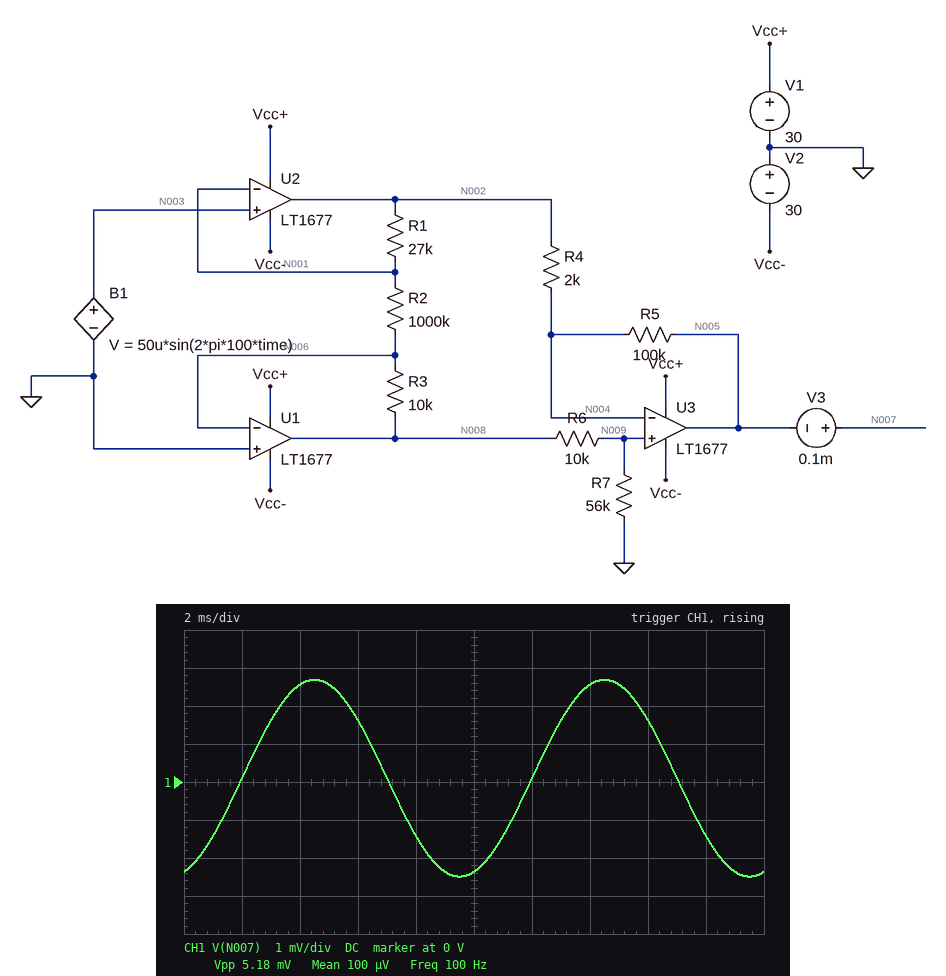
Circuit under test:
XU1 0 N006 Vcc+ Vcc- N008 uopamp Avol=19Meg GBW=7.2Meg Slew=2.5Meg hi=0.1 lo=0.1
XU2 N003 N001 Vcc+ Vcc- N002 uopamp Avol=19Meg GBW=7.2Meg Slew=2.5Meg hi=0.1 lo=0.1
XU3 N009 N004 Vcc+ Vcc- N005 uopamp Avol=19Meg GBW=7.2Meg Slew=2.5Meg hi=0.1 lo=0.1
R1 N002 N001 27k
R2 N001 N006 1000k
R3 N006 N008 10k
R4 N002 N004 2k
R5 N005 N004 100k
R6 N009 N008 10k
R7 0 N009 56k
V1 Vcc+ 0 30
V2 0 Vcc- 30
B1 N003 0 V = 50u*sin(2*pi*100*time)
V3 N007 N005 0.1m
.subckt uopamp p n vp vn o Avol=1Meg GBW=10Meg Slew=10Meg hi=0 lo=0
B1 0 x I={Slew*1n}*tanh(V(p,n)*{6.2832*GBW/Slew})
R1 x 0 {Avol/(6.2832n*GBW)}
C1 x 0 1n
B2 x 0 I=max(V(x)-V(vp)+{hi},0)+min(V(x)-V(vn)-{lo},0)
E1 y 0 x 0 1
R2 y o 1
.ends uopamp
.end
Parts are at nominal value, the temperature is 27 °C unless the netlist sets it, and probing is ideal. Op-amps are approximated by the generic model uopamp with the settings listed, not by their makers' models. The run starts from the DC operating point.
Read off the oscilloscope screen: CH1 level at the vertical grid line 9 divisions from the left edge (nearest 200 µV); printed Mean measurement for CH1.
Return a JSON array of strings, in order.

["-1.4 mV", "100 µV"]
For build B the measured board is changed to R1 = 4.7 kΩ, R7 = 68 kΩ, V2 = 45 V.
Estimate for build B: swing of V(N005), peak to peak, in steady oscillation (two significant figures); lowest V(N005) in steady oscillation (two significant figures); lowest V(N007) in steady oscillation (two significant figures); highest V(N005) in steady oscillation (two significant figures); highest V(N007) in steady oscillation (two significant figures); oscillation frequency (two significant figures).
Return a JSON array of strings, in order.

["5.1 mV", "-2.5 mV", "-2.4 mV", "2.5 mV", "2.6 mV", "100 Hz"]
